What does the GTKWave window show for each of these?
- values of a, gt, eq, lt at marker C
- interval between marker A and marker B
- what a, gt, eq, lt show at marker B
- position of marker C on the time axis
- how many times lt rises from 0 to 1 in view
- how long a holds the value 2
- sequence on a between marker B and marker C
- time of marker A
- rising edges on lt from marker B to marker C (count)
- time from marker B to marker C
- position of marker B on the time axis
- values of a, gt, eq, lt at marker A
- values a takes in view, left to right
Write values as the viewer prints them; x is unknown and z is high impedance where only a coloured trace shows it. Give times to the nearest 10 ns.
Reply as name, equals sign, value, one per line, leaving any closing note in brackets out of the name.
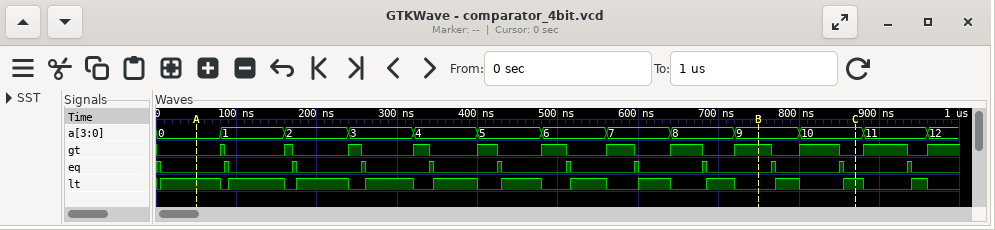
values of a, gt, eq, lt at marker C = a=10, gt=0, eq=0, lt=1
interval between marker A and marker B = 700 ns
what a, gt, eq, lt show at marker B = a=9, gt=1, eq=0, lt=0
position of marker C on the time axis = 870 ns
how many times lt rises from 0 to 1 in view = 12
how long a holds the value 2 = 80 ns
sequence on a between marker B and marker C = 9, 10
time of marker A = 50 ns
rising edges on lt from marker B to marker C = 2
time from marker B to marker C = 120 ns
position of marker B on the time axis = 750 ns
values of a, gt, eq, lt at marker A = a=0, gt=0, eq=0, lt=1
values a takes in view, left to right = 0, 1, 2, 3, 4, 5, 6, 7, 8, 9, 10, 11, 12
